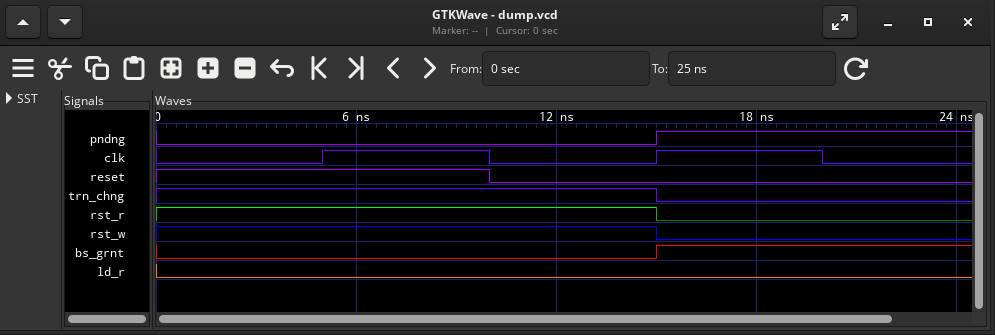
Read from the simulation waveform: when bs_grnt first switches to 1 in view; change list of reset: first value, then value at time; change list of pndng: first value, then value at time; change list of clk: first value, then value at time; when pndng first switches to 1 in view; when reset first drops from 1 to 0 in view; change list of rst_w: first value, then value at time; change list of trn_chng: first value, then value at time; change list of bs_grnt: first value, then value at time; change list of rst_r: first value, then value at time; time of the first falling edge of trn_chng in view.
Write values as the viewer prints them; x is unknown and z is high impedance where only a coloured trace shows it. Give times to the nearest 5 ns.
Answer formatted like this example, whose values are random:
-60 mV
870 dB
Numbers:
15 ns
1, 0 at 10 ns
0, 1 at 15 ns
0, 1 at 5 ns, 0 at 10 ns, 1 at 15 ns, 0 at 20 ns
15 ns
10 ns
1, 0 at 15 ns
1, 0 at 15 ns
0, 1 at 15 ns
1, 0 at 15 ns
15 ns
